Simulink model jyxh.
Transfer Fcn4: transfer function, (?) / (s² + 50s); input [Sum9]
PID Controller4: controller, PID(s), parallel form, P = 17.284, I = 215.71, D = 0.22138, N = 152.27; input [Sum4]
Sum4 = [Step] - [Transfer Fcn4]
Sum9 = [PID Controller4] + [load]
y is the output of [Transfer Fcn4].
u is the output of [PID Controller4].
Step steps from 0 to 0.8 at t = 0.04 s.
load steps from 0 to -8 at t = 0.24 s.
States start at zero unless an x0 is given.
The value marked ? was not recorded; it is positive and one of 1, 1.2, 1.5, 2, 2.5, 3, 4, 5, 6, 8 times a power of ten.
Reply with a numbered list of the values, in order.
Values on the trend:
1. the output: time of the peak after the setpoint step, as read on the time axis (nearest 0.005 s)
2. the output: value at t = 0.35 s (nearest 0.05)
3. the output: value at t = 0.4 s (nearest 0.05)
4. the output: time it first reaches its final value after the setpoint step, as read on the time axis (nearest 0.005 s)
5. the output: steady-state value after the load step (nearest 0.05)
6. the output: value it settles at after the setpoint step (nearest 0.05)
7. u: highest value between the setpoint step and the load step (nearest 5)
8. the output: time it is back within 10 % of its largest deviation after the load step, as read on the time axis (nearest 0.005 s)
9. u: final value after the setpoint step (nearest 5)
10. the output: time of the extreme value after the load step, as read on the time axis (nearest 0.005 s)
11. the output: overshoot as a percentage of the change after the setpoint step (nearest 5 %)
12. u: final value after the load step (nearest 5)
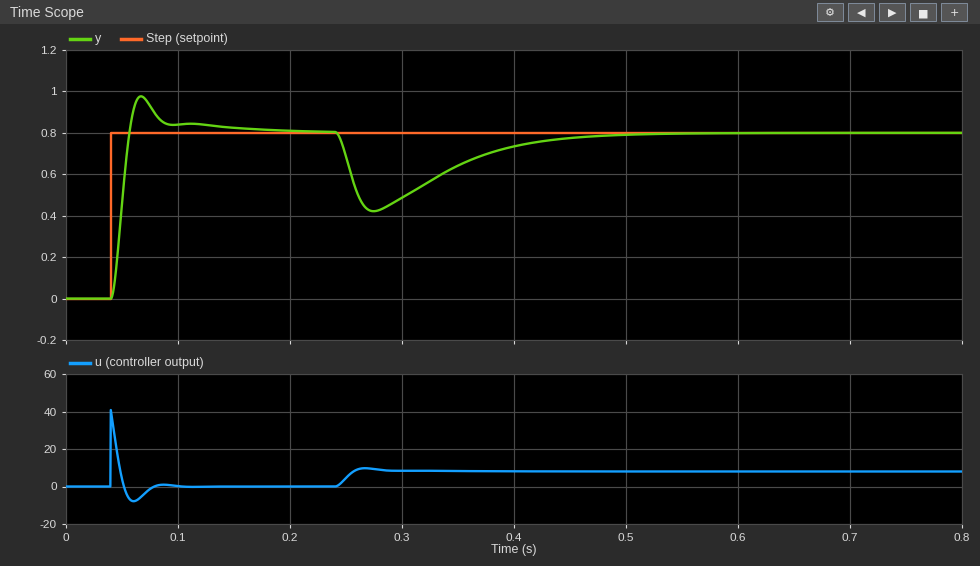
1. 0.065 s
2. 0.65
3. 0.75
4. 0.055 s
5. 0.80
6. 0.80
7. 40
8. 0.430 s
9. 0
10. 0.275 s
11. 20 %
12. 10
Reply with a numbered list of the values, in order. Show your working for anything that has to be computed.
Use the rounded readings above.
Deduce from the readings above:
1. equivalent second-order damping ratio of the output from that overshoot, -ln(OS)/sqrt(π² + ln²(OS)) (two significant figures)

1. ln(0.2) = -1.609; 1.609 / sqrt(9.870 + 2.590) = 0.46
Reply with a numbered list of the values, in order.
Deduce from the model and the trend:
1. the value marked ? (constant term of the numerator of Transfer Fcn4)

1. 400
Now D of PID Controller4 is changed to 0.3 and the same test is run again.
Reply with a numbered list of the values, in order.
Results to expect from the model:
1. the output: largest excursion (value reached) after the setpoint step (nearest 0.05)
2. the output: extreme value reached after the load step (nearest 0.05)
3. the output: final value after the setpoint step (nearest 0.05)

1. 0.95
2. 0.45
3. 0.80
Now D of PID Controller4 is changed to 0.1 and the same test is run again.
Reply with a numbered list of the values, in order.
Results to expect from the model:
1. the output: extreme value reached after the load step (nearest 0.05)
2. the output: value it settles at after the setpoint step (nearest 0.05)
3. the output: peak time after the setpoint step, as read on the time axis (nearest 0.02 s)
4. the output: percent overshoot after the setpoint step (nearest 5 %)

1. 0.35
2. 0.80
3. 0.08 s
4. 35 %
